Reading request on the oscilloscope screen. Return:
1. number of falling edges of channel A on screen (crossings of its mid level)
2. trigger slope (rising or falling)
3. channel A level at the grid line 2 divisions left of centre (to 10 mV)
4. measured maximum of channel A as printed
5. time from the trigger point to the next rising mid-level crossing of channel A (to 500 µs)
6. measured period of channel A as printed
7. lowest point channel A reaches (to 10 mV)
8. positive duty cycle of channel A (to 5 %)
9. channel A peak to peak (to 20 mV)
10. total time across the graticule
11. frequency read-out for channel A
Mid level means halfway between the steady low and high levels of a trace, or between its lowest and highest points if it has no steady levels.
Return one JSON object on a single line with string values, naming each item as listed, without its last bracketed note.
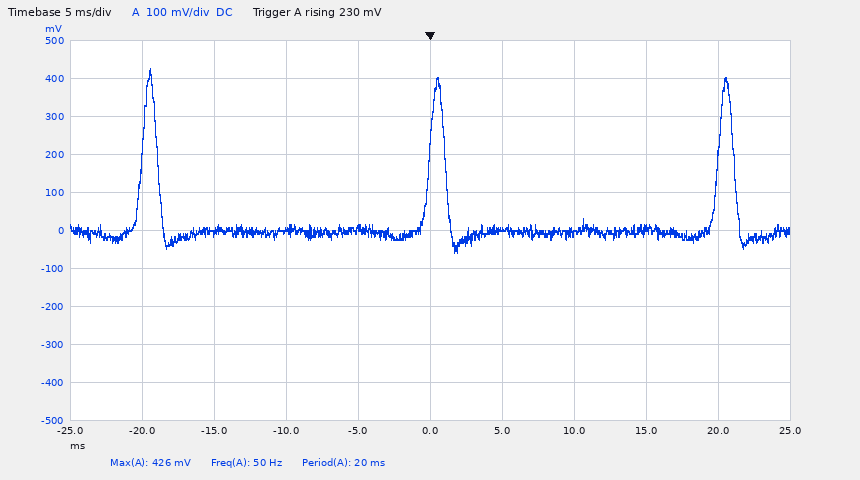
{"number of falling edges of channel A on screen": "3", "trigger slope": "rising", "channel A level at the grid line 2 divisions left of centre": "0 mV", "measured maximum of channel A as printed": "426 mV", "time from the trigger point to the next rising mid-level crossing of channel A": "20.0 ms", "measured period of channel A as printed": "20 ms", "lowest point channel A reaches": "-60 mV", "positive duty cycle of channel A": "5 %", "channel A peak to peak": "480 mV", "total time across the graticule": "50 ms", "frequency read-out for channel A": "50 Hz"}
